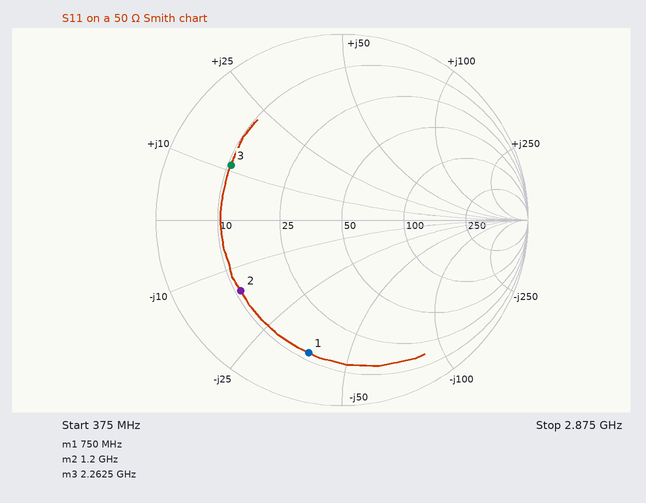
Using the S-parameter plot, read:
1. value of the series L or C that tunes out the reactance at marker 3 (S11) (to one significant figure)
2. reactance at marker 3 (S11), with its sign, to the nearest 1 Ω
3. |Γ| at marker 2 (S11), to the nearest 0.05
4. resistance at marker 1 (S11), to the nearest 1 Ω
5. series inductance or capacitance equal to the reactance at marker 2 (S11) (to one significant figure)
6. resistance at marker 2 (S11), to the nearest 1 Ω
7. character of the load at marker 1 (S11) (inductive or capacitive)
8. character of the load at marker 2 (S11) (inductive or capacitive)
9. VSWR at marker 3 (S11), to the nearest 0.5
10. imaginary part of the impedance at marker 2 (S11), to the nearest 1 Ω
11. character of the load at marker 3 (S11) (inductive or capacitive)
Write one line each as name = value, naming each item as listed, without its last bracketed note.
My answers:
value of the series L or C that tunes out the reactance at marker 3 (S11) = 6 pF
reactance at marker 3 (S11), with its sign, to the nearest 1 Ω = +11 Ω
|Γ| at marker 2 (S11), to the nearest 0.05 = 0.65
resistance at marker 1 (S11), to the nearest 1 Ω = 12 Ω
series inductance or capacitance equal to the reactance at marker 2 (S11) = 9 pF
resistance at marker 2 (S11), to the nearest 1 Ω = 11 Ω
character of the load at marker 1 (S11) = capacitive
character of the load at marker 2 (S11) = capacitive
VSWR at marker 3 (S11), to the nearest 0.5 = 5.0
imaginary part of the impedance at marker 2 (S11), to the nearest 1 Ω = -15 Ω
character of the load at marker 3 (S11) = inductive
